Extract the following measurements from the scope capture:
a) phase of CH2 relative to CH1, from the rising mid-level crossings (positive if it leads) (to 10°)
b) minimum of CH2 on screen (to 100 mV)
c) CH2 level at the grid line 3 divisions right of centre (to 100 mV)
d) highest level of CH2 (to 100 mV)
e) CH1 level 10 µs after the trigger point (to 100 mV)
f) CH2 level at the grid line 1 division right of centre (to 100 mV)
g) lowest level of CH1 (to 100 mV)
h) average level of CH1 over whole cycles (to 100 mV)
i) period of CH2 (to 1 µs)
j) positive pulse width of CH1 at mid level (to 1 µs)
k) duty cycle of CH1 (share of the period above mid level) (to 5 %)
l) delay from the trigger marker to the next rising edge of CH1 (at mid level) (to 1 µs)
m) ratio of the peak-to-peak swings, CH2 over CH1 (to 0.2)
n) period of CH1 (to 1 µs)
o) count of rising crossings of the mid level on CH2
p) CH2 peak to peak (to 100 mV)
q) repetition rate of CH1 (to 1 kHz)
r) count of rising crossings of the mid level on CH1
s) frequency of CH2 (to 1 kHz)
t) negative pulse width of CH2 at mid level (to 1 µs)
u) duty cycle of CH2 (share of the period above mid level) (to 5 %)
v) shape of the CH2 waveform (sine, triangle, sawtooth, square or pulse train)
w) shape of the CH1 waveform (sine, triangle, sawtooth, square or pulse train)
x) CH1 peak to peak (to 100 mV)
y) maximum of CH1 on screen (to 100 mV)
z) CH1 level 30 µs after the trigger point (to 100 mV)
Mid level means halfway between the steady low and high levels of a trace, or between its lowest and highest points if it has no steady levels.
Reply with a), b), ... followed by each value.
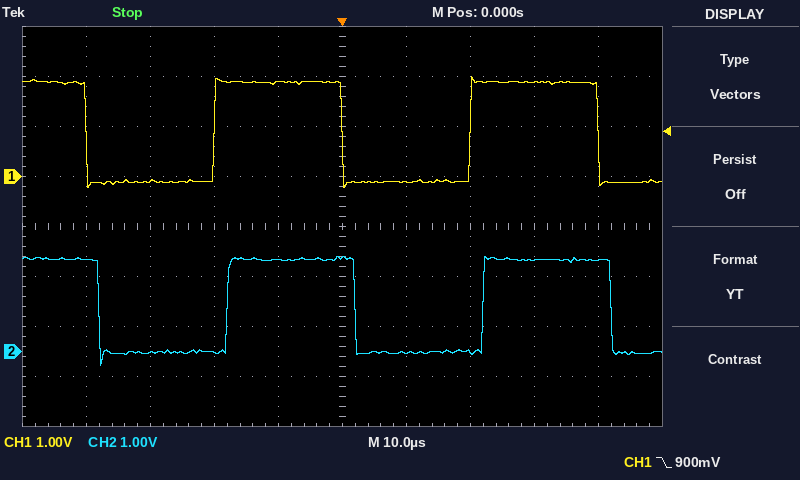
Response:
a) -20°
b) -300 mV
c) 1.8 V
d) 1.9 V
e) -100 mV
f) 0.0 V
g) -200 mV
h) 900 mV
i) 40 µs
j) 20 µs
k) 50 %
l) 20 µs
m) 1.0
n) 40 µs
o) 2
p) 2.2 V
q) 25 kHz
r) 2
s) 25 kHz
t) 20 µs
u) 50 %
v) square
w) square
x) 2.2 V
y) 2.0 V
z) 1.9 V
